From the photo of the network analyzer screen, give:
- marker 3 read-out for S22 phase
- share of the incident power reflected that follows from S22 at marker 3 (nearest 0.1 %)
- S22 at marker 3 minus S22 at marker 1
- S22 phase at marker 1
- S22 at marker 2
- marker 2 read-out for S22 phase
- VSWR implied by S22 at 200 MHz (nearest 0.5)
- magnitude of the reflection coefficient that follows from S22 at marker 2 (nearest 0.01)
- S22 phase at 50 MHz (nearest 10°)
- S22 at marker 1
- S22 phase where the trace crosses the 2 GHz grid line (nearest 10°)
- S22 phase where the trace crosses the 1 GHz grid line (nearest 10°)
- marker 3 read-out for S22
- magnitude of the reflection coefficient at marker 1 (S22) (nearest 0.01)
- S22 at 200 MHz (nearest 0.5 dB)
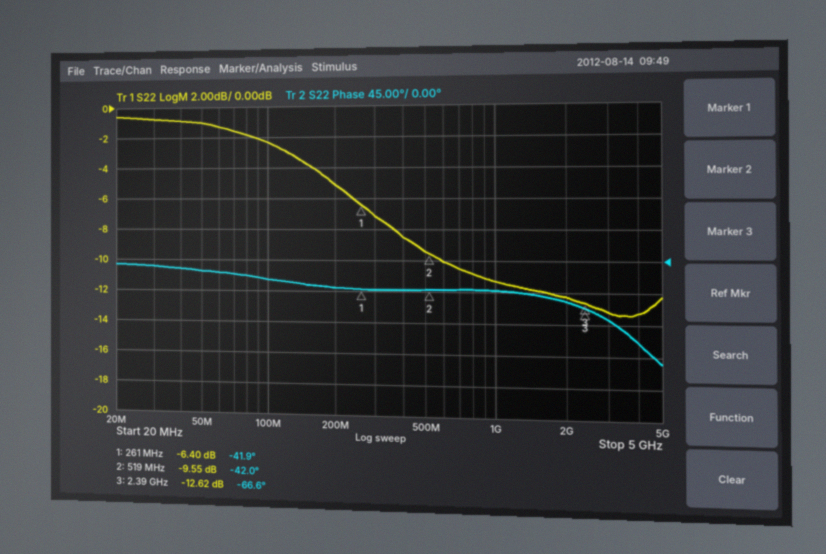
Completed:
-66.6°
5.5 %
-6.22 dB
-41.9°
-9.55 dB
-42.0°
3.5
0.33
-20°
-6.40 dB
-60°
-40°
-12.62 dB
0.48
-5.0 dB
